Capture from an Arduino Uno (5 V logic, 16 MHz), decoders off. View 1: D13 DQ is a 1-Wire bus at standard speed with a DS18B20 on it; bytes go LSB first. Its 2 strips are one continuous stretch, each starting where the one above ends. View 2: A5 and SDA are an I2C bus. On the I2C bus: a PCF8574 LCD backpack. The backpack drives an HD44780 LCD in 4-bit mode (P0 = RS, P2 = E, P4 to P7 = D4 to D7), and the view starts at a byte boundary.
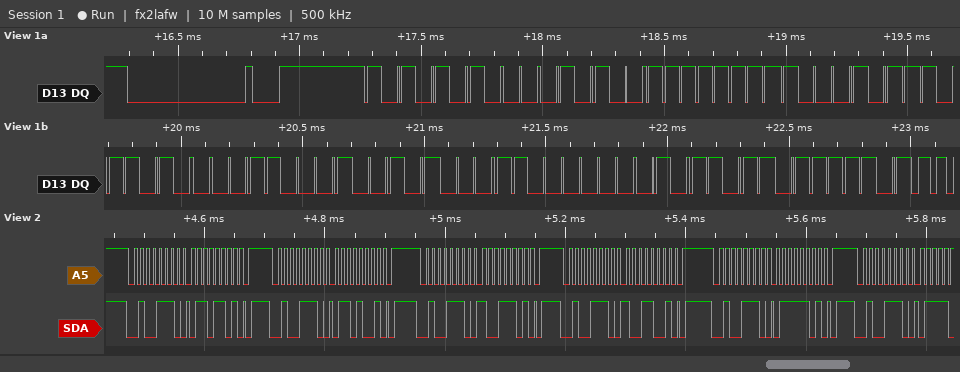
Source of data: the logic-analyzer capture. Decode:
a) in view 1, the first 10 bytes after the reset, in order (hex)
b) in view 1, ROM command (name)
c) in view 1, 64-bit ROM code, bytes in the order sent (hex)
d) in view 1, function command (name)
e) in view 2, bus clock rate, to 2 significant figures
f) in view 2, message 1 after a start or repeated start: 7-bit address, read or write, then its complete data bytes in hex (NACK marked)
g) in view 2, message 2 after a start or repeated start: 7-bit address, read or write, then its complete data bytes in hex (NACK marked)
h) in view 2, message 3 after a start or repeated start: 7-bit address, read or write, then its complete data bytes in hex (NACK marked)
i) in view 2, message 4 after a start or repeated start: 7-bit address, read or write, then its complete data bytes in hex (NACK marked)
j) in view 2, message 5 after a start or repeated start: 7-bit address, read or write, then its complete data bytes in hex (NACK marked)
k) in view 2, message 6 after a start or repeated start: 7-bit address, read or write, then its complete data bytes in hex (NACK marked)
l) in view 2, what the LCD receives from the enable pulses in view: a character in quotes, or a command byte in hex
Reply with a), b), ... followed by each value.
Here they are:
a) 55 28 FF D1 2D 8C 14 03 DA BE
b) Match ROM
c) 28 FF D1 2D 8C 14 03 DA
d) Read Scratchpad
e) 100 kHz
f) 0x27 write: 6D
g) 0x27 write: 69
h) 0x27 write: 9D
i) 0x27 write: 99
j) 0x27 write: 7D
k) 0x27 write
l) 'i'
